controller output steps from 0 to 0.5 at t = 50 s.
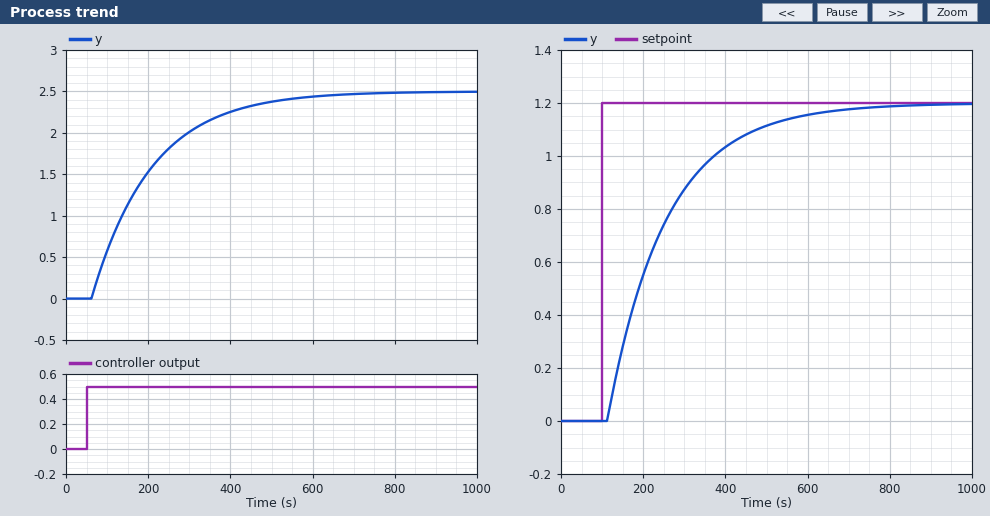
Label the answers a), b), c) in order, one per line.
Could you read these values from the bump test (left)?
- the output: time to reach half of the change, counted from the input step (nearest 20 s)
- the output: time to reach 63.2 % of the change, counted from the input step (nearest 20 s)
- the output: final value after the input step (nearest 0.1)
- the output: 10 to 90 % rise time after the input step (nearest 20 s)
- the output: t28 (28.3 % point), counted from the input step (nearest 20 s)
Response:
a) 120 s
b) 160 s
c) 2.5
d) 320 s
e) 60 s
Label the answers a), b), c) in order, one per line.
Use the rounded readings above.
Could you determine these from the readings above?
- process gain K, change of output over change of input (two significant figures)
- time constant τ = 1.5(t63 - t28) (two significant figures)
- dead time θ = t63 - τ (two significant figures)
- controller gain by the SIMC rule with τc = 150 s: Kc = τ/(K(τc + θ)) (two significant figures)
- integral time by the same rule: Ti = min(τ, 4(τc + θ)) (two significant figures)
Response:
a) 5.0
b) 150 s
c) 10 s
d) 0.19
e) 150 s
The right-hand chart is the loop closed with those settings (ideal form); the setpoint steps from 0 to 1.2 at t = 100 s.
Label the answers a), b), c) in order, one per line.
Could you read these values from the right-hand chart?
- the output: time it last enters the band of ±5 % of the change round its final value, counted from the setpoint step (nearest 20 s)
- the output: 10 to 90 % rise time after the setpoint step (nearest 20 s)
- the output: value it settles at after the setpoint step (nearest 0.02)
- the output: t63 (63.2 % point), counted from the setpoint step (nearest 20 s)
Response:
a) 460 s
b) 320 s
c) 1.20
d) 160 s
